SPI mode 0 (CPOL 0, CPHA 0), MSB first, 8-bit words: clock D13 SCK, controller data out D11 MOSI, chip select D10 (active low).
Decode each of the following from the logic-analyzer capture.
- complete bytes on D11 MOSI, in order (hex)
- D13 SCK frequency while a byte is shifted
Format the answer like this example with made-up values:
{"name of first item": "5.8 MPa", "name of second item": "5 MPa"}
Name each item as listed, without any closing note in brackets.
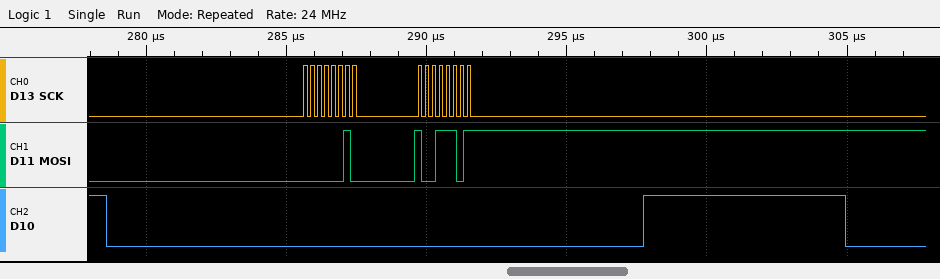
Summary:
{"complete bytes on D11 MOSI, in order": "02 9D", "D13 SCK frequency while a byte is shifted": "4 MHz"}
